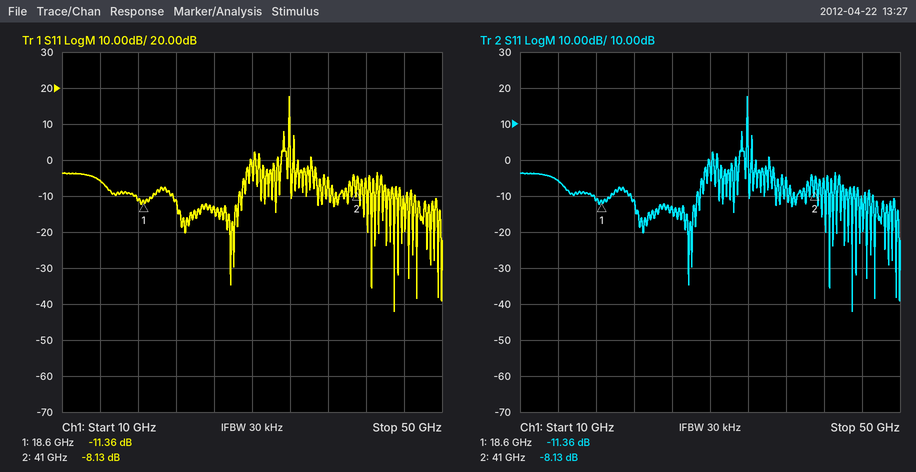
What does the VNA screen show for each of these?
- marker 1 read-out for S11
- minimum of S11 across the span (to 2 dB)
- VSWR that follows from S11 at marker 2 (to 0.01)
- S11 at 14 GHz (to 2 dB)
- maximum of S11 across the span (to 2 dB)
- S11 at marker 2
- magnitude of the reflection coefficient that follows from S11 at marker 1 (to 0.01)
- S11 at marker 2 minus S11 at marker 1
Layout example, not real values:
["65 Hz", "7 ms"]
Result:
["-11.36 dB", "-42 dB", "2.29", "-6 dB", "18 dB", "-8.13 dB", "0.27", "3.23 dB"]
